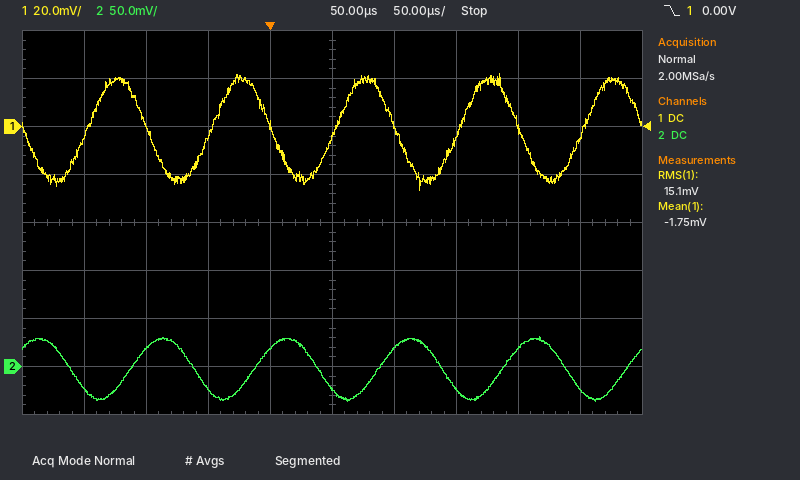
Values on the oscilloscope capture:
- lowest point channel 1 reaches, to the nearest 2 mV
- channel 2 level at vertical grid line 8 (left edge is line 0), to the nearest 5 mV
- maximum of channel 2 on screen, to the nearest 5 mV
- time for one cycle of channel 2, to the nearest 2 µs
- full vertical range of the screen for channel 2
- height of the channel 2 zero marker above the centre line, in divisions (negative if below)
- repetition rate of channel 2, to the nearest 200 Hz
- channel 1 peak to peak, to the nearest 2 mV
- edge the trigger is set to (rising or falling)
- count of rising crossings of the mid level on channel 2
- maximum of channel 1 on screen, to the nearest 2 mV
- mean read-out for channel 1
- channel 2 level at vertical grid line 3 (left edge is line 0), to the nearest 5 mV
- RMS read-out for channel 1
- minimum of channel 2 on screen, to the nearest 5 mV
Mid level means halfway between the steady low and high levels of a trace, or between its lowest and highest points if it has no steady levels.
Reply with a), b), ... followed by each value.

a) -26 mV
b) 20 mV
c) 30 mV
d) 100 µs
e) 400 mV
f) -3.0 div
g) 10.0 kHz
h) 48 mV
i) falling
j) 5
k) 22 mV
l) -1.75 mV
m) -25 mV
n) 15.1 mV
o) -35 mV
